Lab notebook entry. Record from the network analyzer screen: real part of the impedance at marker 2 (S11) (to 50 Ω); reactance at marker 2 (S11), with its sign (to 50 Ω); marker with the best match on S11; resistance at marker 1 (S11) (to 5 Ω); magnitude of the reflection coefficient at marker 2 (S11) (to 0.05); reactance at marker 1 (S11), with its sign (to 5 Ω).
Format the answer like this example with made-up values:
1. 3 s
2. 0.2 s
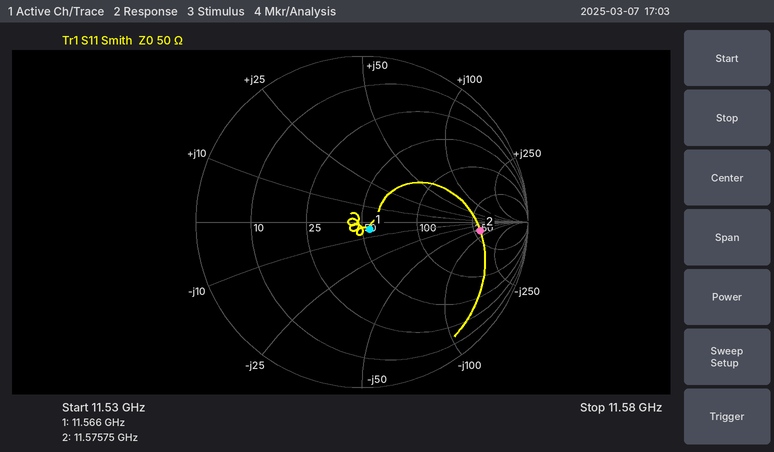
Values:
1. 300 Ω
2. -50 Ω
3. marker 1
4. 55 Ω
5. 0.70
6. -5 Ω
